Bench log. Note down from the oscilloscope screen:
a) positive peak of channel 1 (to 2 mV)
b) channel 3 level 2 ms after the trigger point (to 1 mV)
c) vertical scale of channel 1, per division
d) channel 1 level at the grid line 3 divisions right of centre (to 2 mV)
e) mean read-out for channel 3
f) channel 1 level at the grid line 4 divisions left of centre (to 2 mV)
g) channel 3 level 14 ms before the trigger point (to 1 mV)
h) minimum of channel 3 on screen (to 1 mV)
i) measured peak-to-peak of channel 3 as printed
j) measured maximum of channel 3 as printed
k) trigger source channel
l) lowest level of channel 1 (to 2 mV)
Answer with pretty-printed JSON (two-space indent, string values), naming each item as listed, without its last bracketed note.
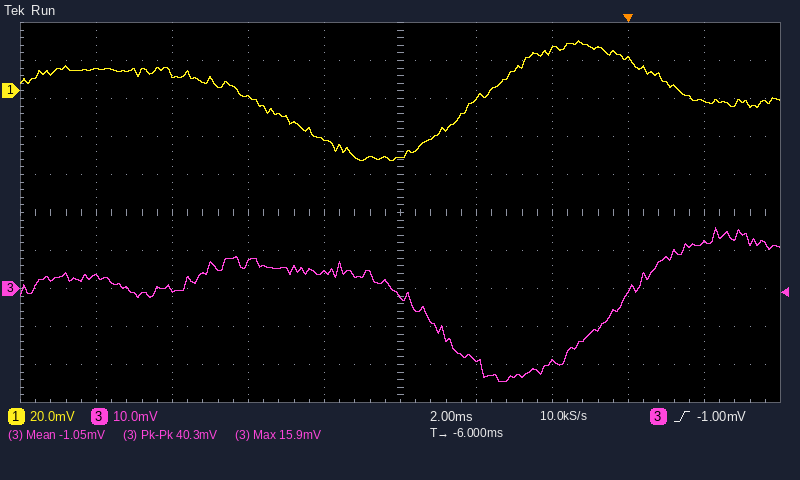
{
  "positive peak of channel 1": "26 mV",
  "channel 3 level 2 ms after the trigger point": "12 mV",
  "vertical scale of channel 1, per division": "20 mV",
  "channel 1 level at the grid line 3 divisions right of centre": "16 mV",
  "mean read-out for channel 3": "-1.05 mV",
  "channel 1 level at the grid line 4 divisions left of centre": "12 mV",
  "channel 3 level 14 ms before the trigger point": "3 mV",
  "minimum of channel 3 on screen": "-24 mV",
  "measured peak-to-peak of channel 3 as printed": "40.3 mV",
  "measured maximum of channel 3 as printed": "15.9 mV",
  "trigger source channel": "channel 3",
  "lowest level of channel 1": "-36 mV"
}
